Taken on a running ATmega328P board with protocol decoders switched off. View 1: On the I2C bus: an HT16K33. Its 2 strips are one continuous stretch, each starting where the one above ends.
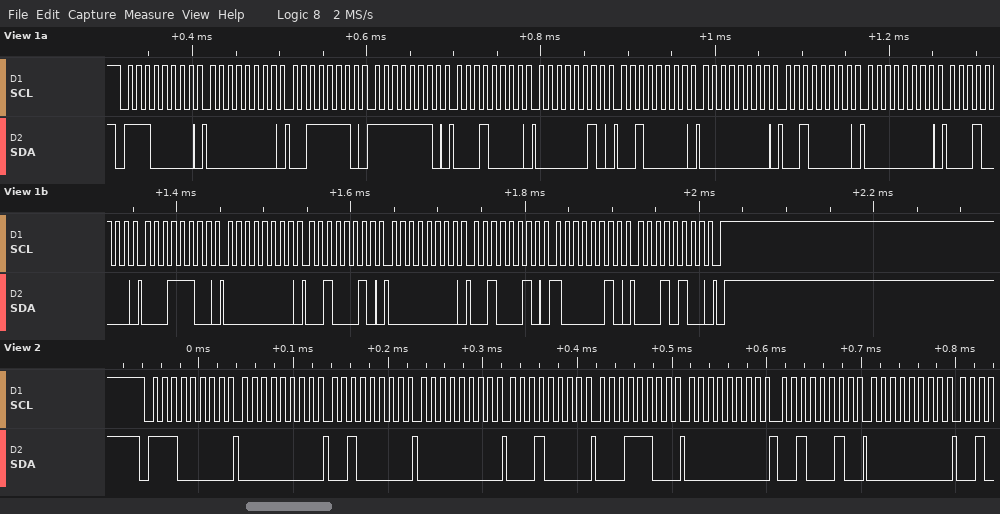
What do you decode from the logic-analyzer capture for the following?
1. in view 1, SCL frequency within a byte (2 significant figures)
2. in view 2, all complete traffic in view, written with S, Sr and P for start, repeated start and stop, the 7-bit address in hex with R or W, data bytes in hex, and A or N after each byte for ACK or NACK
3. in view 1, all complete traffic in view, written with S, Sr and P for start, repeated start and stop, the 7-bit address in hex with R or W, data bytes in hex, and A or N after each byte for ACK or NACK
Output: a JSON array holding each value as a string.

["100 kHz", "S 70W A 00 A 20 A 00 A 10 A 1C A 00 A 22 A 00 A", "S 70W A 00 A 3E A FE A 10 A 02 A 20 A 00 A 20 A 00 A 10 A 1C A 00 A 22 A 00 A 22 A 82 A 14 A P"]
